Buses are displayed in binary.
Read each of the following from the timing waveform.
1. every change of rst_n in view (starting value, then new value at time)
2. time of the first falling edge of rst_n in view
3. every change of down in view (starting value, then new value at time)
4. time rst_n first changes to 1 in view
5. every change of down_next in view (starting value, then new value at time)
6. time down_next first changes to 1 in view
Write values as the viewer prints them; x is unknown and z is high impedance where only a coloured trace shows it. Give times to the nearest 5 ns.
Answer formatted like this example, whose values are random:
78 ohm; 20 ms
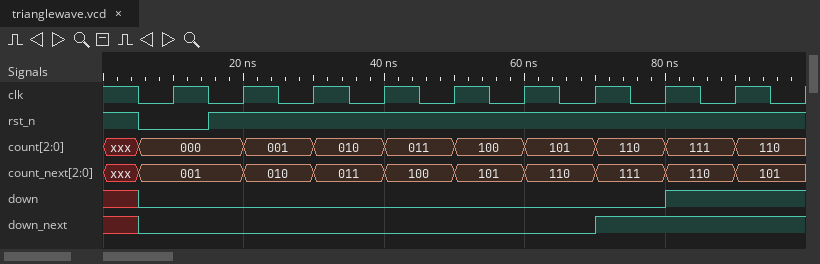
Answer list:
1, 0 at 5 ns, 1 at 15 ns; 5 ns; x, 0 at 5 ns, 1 at 80 ns; 15 ns; x, 0 at 5 ns, 1 at 70 ns; 70 ns
